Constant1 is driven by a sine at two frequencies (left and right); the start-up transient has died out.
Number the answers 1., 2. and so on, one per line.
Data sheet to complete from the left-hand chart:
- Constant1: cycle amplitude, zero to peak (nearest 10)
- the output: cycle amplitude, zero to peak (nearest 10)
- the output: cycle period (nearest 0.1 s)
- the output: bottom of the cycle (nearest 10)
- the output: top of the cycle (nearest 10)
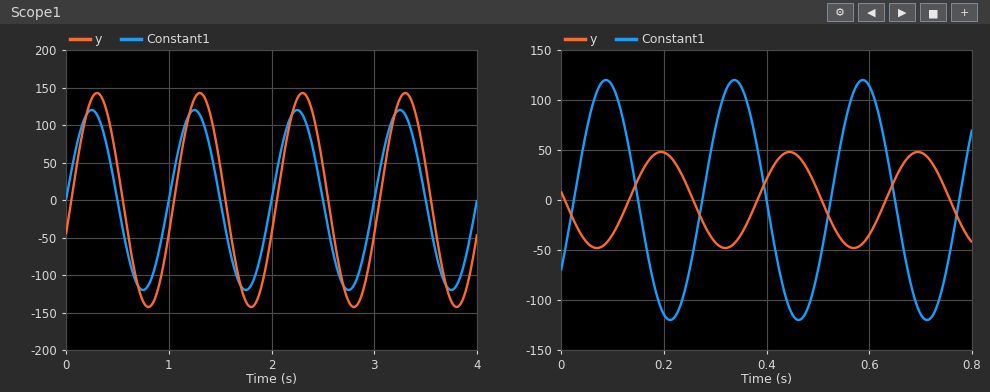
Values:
1. 120
2. 140
3. 1.0 s
4. -140
5. 140
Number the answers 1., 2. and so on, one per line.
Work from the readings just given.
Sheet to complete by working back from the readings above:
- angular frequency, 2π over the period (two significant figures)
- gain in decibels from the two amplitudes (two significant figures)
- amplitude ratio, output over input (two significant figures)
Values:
1. 6.3 rad/s
2. 1.3 dB
3. 1.2
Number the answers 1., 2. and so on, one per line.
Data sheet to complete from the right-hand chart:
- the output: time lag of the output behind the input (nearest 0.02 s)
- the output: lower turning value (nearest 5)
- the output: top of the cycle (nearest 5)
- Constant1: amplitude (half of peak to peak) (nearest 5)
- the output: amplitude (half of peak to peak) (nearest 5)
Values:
1. 0.10 s
2. -50
3. 50
4. 120
5. 50
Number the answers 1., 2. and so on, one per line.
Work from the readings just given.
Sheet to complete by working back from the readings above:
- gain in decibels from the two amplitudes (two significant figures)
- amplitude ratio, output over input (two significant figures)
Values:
1. -7.6 dB
2. 0.42
